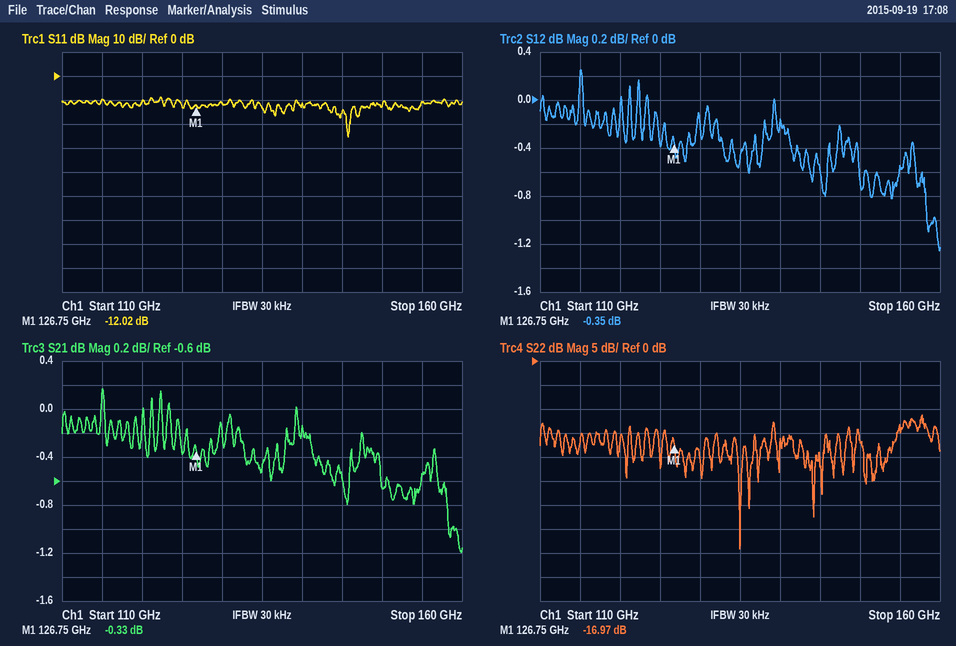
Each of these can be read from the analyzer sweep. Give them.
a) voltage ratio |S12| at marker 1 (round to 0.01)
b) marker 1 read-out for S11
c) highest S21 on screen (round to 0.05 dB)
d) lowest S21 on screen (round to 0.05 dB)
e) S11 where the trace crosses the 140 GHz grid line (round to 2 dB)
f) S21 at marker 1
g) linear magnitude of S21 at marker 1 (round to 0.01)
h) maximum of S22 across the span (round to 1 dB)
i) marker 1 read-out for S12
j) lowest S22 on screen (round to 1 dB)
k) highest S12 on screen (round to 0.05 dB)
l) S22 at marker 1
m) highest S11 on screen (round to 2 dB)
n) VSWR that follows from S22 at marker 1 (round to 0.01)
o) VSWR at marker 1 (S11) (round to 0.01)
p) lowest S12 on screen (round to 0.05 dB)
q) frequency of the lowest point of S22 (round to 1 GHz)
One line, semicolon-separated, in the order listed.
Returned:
0.96; -12.02 dB; 0.15 dB; -1.20 dB; -12 dB; -0.33 dB; 0.96; -11 dB; -0.35 dB; -39 dB; 0.25 dB; -16.97 dB; -8 dB; 1.33; 1.67; -1.25 dB; 135 GHz
